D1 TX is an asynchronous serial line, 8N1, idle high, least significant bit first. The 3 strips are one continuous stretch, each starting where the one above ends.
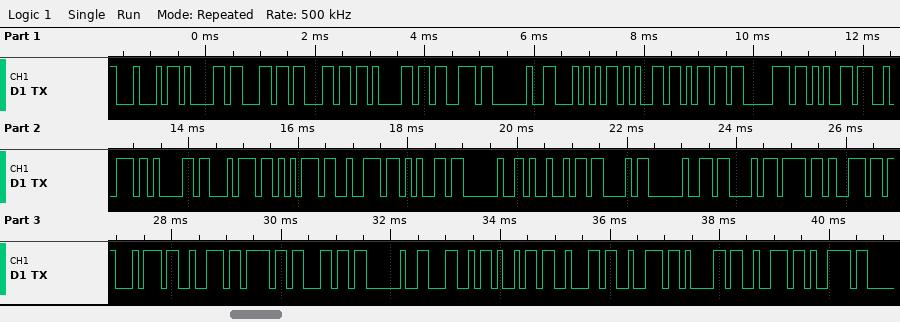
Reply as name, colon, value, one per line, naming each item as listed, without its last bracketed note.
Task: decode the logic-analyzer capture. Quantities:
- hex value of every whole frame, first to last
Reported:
hex value of every whole frame, first to last: 44 61 6C 6C 61 73 20 54 65 6D 70 65 72 61 74 75 72 65 20 49 43 20 43 6F 6E 74 72 6F 6C 20 4C 69 62 72 61 72 79
